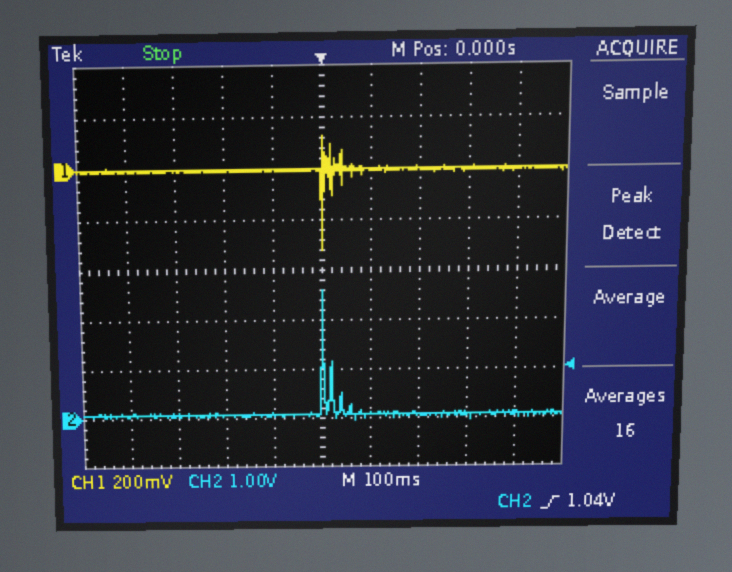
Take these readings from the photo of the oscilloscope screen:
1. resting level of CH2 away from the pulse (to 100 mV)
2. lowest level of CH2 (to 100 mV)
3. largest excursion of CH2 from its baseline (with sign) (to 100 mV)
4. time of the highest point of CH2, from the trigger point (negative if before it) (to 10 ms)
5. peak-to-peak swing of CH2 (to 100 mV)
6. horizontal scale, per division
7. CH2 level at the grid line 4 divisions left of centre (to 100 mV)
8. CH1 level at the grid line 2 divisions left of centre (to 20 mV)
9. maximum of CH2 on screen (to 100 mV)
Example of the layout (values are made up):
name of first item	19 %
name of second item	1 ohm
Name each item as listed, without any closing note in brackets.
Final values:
resting level of CH2 away from the pulse	100 mV
lowest level of CH2	0.0 V
largest excursion of CH2 from its baseline (with sign)	+2.5 V
time of the highest point of CH2, from the trigger point (negative if before it)	0 ms
peak-to-peak swing of CH2	2.6 V
horizontal scale, per division	100 ms
CH2 level at the grid line 4 divisions left of centre	100 mV
CH1 level at the grid line 2 divisions left of centre	0 mV
maximum of CH2 on screen	2.6 V
